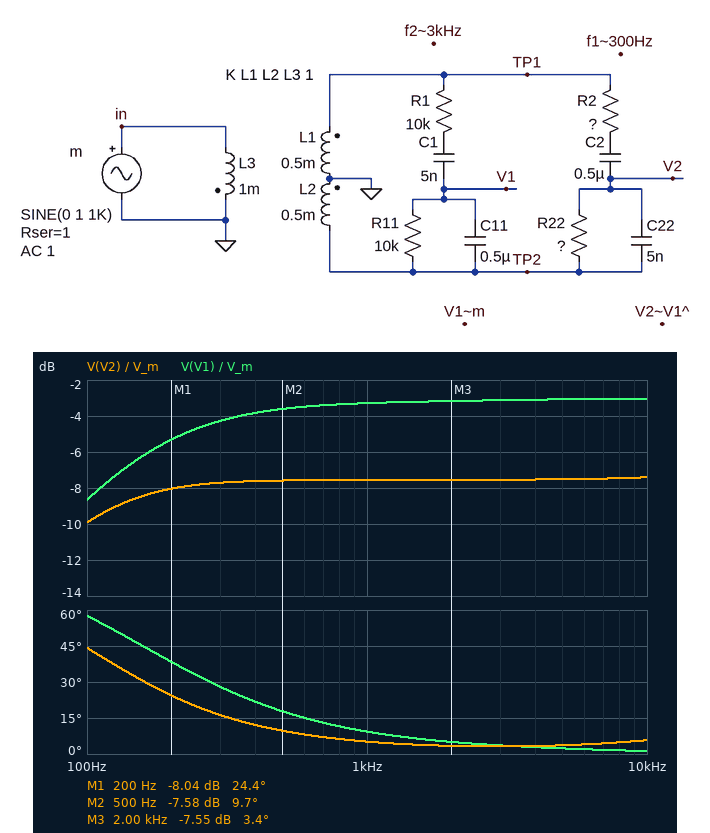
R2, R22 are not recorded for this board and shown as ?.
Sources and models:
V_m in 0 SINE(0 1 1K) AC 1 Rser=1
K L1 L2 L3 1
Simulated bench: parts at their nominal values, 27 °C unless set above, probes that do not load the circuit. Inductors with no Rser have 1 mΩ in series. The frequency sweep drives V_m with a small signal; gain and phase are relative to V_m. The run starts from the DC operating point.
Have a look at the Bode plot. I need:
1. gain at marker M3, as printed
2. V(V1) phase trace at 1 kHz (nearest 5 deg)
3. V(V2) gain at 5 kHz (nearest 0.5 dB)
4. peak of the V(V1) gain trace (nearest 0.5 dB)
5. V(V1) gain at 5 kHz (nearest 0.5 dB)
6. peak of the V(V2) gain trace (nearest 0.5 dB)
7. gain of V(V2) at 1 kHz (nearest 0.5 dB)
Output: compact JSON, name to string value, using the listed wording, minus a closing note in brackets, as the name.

{"gain at marker M3, as printed": "-7.55 dB", "V(V1) phase trace at 1 kHz": "10 deg", "V(V2) gain at 5 kHz": "-7.5 dB", "peak of the V(V1) gain trace": "-3.0 dB", "V(V1) gain at 5 kHz": "-3.0 dB", "peak of the V(V2) gain trace": "-7.5 dB", "gain of V(V2) at 1 kHz": "-7.5 dB"}
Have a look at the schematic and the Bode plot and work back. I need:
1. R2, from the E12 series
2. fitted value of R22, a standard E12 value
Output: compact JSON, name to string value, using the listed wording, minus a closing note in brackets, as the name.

{"R2, from the E12 series": "2.2 kΩ", "fitted value of R22, a standard E12 value": "560 Ω"}
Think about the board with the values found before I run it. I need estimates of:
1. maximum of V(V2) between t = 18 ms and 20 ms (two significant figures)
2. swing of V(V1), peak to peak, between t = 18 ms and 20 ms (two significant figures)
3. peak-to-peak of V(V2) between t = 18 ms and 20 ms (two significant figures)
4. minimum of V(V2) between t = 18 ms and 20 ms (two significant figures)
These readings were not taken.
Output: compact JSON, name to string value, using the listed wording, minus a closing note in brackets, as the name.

{"maximum of V(V2) between t = 18 ms and 20 ms": "420 mV", "swing of V(V1), peak to peak, between t = 18 ms and 20 ms": "1.4 V", "peak-to-peak of V(V2) between t = 18 ms and 20 ms": "840 mV", "minimum of V(V2) between t = 18 ms and 20 ms": "-420 mV"}
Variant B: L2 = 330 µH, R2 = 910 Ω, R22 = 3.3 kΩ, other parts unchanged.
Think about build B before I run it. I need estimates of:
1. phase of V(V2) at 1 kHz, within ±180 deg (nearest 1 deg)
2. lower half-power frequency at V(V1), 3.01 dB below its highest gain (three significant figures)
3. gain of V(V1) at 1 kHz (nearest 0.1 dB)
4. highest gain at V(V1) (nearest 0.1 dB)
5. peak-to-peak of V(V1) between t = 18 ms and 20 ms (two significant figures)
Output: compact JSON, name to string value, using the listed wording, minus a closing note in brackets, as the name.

{"phase of V(V2) at 1 kHz, within ±180 deg": "-164 deg", "lower half-power frequency at V(V1), 3.01 dB below its highest gain": "166 Hz", "gain of V(V1) at 1 kHz": "-5.1 dB", "highest gain at V(V1)": "-4.8 dB", "peak-to-peak of V(V1) between t = 18 ms and 20 ms": "1.1 V"}
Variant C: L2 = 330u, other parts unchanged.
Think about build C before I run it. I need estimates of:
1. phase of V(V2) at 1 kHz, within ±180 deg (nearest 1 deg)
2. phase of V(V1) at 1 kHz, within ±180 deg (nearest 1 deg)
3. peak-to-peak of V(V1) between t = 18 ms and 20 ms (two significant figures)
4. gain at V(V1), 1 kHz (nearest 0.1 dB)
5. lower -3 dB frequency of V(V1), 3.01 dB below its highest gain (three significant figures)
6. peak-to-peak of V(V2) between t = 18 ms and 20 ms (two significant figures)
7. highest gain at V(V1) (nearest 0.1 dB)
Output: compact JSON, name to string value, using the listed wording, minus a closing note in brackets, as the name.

{"phase of V(V2) at 1 kHz, within ±180 deg": "4 deg", "phase of V(V1) at 1 kHz, within ±180 deg": "9 deg", "peak-to-peak of V(V1) between t = 18 ms and 20 ms": "1.1 V", "gain at V(V1), 1 kHz": "-5.1 dB", "lower -3 dB frequency of V(V1), 3.01 dB below its highest gain": "166 Hz", "peak-to-peak of V(V2) between t = 18 ms and 20 ms": "630 mV", "highest gain at V(V1)": "-4.8 dB"}
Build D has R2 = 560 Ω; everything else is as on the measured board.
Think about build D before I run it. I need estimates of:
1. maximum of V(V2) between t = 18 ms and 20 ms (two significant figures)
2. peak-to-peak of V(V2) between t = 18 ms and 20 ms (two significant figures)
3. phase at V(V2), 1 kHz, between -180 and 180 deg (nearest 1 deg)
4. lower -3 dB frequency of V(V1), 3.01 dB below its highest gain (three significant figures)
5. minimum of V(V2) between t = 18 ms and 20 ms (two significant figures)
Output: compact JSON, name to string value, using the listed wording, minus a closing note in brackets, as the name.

{"maximum of V(V2) between t = 18 ms and 20 ms": "180 mV", "peak-to-peak of V(V2) between t = 18 ms and 20 ms": "370 mV", "phase at V(V2), 1 kHz, between -180 and 180 deg": "-65 deg", "lower -3 dB frequency of V(V1), 3.01 dB below its highest gain": "165 Hz", "minimum of V(V2) between t = 18 ms and 20 ms": "-180 mV"}
